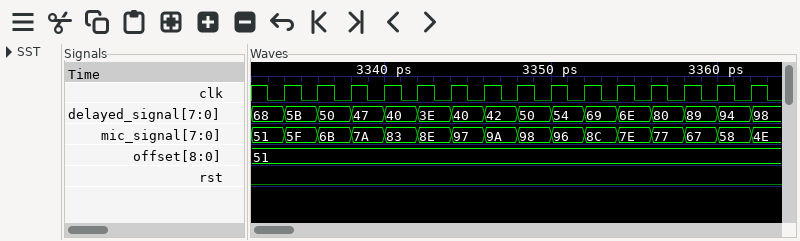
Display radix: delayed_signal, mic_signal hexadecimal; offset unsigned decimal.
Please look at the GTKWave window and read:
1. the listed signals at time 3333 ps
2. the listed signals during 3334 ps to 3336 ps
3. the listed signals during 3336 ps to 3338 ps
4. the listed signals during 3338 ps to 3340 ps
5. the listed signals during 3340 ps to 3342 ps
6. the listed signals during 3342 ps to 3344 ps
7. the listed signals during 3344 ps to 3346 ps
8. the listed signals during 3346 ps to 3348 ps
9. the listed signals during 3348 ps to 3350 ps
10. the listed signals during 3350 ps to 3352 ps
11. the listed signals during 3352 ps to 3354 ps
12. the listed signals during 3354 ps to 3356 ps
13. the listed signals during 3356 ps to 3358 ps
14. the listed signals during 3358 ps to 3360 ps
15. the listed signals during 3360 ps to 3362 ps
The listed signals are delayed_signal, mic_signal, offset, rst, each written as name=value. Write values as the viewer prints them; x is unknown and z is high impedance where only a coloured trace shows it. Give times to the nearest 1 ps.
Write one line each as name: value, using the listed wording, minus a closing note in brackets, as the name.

the listed signals at time 3333 ps: delayed_signal=68, mic_signal=51, offset=51, rst=0
the listed signals during 3334 ps to 3336 ps: delayed_signal=5B, mic_signal=5F, offset=51, rst=0
the listed signals during 3336 ps to 3338 ps: delayed_signal=50, mic_signal=6B, offset=51, rst=0
the listed signals during 3338 ps to 3340 ps: delayed_signal=47, mic_signal=7A, offset=51, rst=0
the listed signals during 3340 ps to 3342 ps: delayed_signal=40, mic_signal=83, offset=51, rst=0
the listed signals during 3342 ps to 3344 ps: delayed_signal=3E, mic_signal=8E, offset=51, rst=0
the listed signals during 3344 ps to 3346 ps: delayed_signal=40, mic_signal=97, offset=51, rst=0
the listed signals during 3346 ps to 3348 ps: delayed_signal=42, mic_signal=9A, offset=51, rst=0
the listed signals during 3348 ps to 3350 ps: delayed_signal=50, mic_signal=98, offset=51, rst=0
the listed signals during 3350 ps to 3352 ps: delayed_signal=54, mic_signal=96, offset=51, rst=0
the listed signals during 3352 ps to 3354 ps: delayed_signal=69, mic_signal=8C, offset=51, rst=0
the listed signals during 3354 ps to 3356 ps: delayed_signal=6E, mic_signal=7E, offset=51, rst=0
the listed signals during 3356 ps to 3358 ps: delayed_signal=80, mic_signal=77, offset=51, rst=0
the listed signals during 3358 ps to 3360 ps: delayed_signal=89, mic_signal=67, offset=51, rst=0
the listed signals during 3360 ps to 3362 ps: delayed_signal=94, mic_signal=58, offset=51, rst=0
